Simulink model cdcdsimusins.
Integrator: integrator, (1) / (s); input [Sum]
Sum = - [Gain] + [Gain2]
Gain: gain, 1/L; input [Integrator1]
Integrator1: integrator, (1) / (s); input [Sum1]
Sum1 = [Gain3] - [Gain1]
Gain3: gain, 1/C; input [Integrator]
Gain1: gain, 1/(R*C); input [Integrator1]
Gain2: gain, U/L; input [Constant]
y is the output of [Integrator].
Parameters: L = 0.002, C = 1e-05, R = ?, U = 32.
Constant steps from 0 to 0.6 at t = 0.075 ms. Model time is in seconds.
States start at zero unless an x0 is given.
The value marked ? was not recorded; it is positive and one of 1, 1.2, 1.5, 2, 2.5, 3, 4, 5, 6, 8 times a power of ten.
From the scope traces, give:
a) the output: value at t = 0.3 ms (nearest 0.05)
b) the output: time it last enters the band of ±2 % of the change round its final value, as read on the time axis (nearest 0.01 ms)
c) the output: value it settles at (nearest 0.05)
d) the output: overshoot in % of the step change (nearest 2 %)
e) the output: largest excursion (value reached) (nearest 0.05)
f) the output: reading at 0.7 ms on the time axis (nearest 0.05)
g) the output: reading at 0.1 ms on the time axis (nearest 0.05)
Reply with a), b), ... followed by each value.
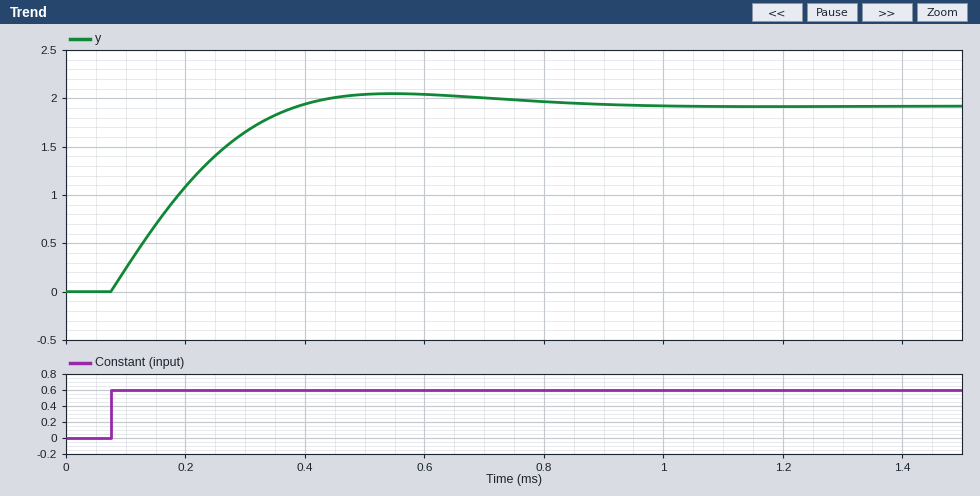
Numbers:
a) 1.65
b) 0.82 ms
c) 1.90
d) 6 %
e) 2.05
f) 2.00
g) 0.25
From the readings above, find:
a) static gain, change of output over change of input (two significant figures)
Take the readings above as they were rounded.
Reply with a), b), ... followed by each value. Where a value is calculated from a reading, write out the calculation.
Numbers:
a) (1.9 - 0) / (0.6 - 0) = 3.2
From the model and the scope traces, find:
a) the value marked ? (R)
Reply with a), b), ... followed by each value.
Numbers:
a) 10
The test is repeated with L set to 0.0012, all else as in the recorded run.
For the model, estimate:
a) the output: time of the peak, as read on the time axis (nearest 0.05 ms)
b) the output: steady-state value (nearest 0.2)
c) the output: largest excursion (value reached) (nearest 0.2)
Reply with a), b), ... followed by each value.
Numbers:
a) 0.35 ms
b) 2.0
c) 2.4
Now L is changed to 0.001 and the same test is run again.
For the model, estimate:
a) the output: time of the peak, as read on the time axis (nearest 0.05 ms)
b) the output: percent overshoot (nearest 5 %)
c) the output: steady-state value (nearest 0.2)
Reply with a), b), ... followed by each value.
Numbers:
a) 0.30 ms
b) 30 %
c) 2.0
